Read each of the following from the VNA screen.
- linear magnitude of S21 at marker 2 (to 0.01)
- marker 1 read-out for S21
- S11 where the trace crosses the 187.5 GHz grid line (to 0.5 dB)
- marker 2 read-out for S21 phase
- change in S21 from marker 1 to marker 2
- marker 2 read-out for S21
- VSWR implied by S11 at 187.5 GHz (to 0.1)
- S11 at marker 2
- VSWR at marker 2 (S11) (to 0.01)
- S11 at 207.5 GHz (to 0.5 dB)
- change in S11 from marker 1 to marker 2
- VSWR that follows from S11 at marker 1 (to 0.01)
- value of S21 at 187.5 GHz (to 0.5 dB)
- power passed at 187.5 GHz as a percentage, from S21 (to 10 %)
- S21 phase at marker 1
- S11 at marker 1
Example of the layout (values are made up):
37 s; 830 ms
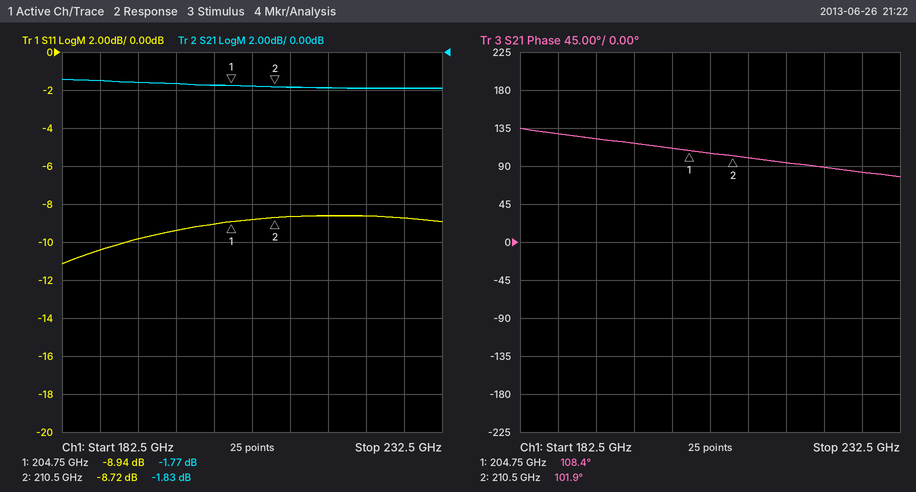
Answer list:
0.81; -1.77 dB; -10.5 dB; 101.9°; -0.06 dB; -1.83 dB; 1.9; -8.72 dB; 2.16; -9.0 dB; 0.22 dB; 2.11; -1.5 dB; 70 %; 108.4°; -8.94 dB
